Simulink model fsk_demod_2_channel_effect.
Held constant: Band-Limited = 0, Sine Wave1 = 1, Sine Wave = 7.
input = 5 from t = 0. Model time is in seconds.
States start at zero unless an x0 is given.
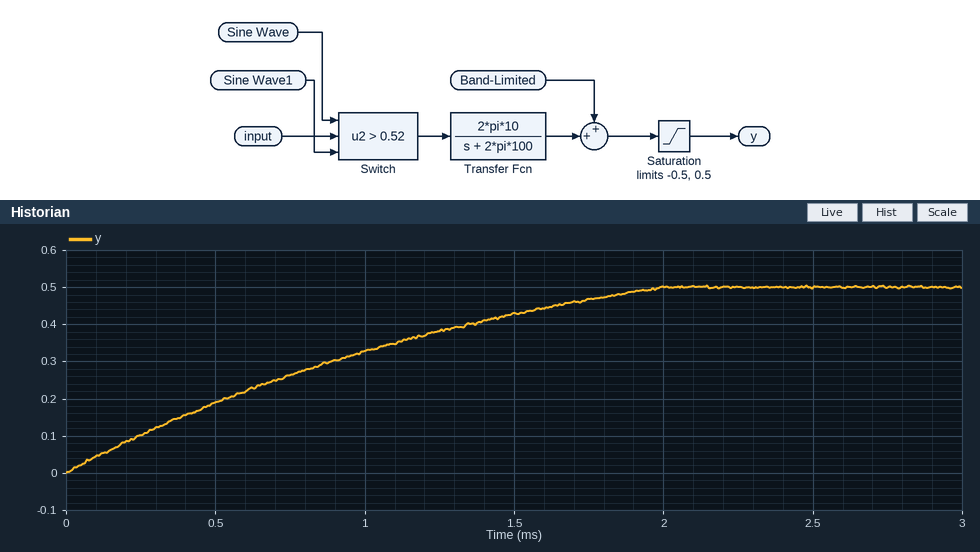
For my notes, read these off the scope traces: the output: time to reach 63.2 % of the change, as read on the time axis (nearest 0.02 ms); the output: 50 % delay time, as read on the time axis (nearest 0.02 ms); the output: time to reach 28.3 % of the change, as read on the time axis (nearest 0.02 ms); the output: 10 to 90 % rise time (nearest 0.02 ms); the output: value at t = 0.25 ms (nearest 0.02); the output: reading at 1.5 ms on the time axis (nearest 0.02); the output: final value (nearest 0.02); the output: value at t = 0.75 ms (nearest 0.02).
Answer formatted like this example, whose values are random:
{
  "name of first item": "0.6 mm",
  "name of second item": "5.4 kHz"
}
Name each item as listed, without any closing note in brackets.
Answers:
{
  "the output: time to reach 63.2 % of the change, as read on the time axis": "0.96 ms",
  "the output: 50 % delay time, as read on the time axis": "0.70 ms",
  "the output: time to reach 28.3 % of the change, as read on the time axis": "0.36 ms",
  "the output: 10 to 90 % rise time": "1.52 ms",
  "the output: value at t = 0.25 ms": "0.10",
  "the output: reading at 1.5 ms on the time axis": "0.42",
  "the output: final value": "0.50",
  "the output: value at t = 0.75 ms": "0.26"
}
